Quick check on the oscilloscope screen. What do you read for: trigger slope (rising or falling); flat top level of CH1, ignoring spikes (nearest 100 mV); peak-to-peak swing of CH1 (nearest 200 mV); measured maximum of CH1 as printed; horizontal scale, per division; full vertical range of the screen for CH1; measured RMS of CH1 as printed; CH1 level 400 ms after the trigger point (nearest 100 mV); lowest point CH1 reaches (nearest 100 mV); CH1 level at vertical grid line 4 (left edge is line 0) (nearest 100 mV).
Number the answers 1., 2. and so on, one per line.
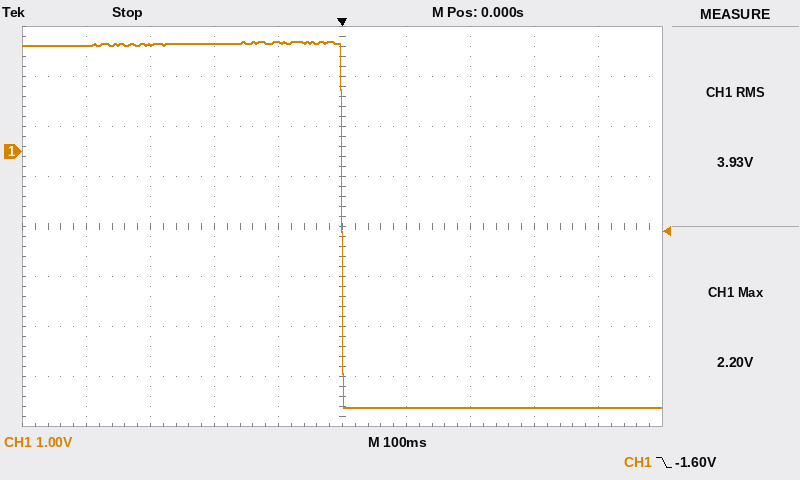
1. falling
2. 2.2 V
3. 7.4 V
4. 2.20 V
5. 100 ms
6. 8 V
7. 3.93 V
8. -5.1 V
9. -5.1 V
10. 2.2 V
